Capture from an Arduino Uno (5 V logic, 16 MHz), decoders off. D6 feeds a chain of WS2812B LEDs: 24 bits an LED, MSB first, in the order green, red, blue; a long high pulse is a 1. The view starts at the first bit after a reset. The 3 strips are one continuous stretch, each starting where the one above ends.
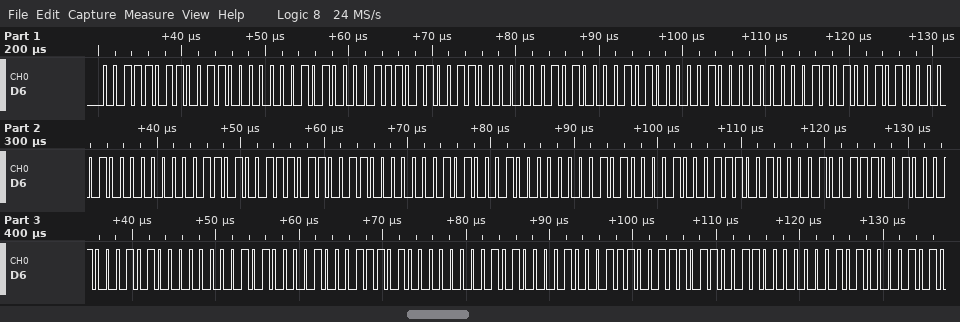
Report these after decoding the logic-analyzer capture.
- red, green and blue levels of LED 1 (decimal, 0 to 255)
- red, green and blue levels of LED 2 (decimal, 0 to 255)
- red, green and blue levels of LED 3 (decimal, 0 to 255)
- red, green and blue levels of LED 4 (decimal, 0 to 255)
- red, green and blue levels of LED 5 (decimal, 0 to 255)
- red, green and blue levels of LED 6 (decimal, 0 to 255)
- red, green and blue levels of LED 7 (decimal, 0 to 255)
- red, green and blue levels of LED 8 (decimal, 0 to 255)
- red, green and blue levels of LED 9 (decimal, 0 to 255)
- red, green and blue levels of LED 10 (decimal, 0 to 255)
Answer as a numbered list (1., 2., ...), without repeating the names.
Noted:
1. 48, 59, 20
2. 48, 59, 20
3. 32, 40, 13
4. 32, 40, 13
5. 48, 59, 20
6. 40, 64, 71
7. 57, 33, 17
8. 40, 64, 71
9. 40, 64, 71
10. 48, 59, 20
